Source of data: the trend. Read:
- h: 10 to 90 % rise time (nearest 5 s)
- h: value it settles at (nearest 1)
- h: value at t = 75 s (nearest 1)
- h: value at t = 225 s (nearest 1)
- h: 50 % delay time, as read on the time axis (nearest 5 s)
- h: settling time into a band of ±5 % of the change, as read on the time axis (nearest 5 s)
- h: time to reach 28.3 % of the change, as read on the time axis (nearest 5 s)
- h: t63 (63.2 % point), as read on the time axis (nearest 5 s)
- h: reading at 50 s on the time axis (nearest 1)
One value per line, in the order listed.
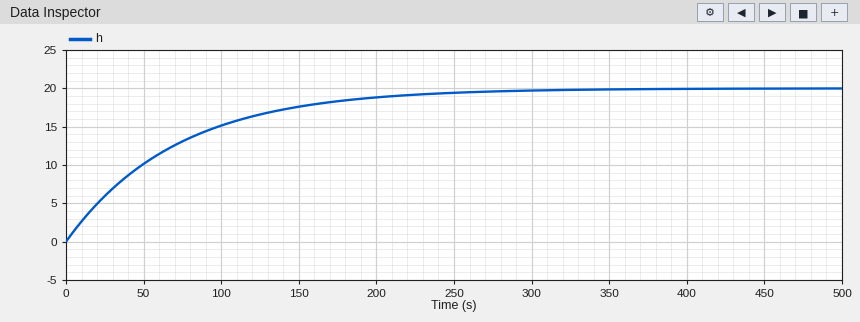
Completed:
155 s
20
13
19
50 s
210 s
25 s
70 s
10
